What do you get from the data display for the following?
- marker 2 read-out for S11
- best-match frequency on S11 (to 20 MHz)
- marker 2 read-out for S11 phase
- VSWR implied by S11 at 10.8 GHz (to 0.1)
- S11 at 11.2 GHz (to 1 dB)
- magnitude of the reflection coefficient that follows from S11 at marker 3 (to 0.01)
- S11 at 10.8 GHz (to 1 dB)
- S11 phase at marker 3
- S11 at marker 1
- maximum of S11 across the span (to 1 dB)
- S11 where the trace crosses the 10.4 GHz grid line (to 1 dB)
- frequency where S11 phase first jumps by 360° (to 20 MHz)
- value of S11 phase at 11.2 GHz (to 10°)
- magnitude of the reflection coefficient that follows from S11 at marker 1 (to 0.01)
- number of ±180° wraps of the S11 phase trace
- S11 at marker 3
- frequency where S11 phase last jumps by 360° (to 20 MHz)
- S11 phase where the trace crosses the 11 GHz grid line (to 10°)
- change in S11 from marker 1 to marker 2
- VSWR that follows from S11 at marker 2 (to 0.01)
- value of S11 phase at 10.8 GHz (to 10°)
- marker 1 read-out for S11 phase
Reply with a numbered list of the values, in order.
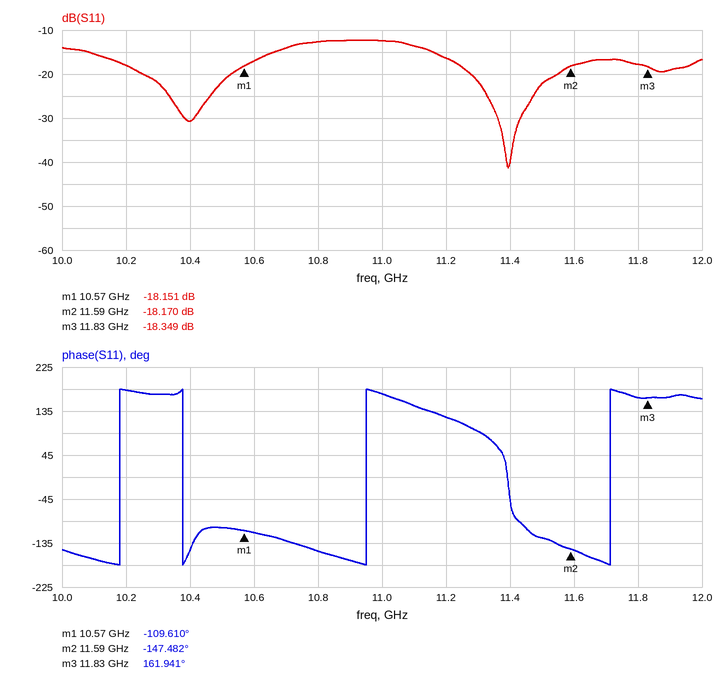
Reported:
1. -18.170 dB
2. 11.40 GHz
3. -147.482°
4. 1.6
5. -16 dB
6. 0.12
7. -13 dB
8. 161.941°
9. -18.151 dB
10. -12 dB
11. -31 dB
12. 10.18 GHz
13. 120°
14. 0.12
15. 4
16. -18.349 dB
17. 11.72 GHz
18. 170°
19. -0.019 dB
20. 1.28
21. -150°
22. -109.610°
